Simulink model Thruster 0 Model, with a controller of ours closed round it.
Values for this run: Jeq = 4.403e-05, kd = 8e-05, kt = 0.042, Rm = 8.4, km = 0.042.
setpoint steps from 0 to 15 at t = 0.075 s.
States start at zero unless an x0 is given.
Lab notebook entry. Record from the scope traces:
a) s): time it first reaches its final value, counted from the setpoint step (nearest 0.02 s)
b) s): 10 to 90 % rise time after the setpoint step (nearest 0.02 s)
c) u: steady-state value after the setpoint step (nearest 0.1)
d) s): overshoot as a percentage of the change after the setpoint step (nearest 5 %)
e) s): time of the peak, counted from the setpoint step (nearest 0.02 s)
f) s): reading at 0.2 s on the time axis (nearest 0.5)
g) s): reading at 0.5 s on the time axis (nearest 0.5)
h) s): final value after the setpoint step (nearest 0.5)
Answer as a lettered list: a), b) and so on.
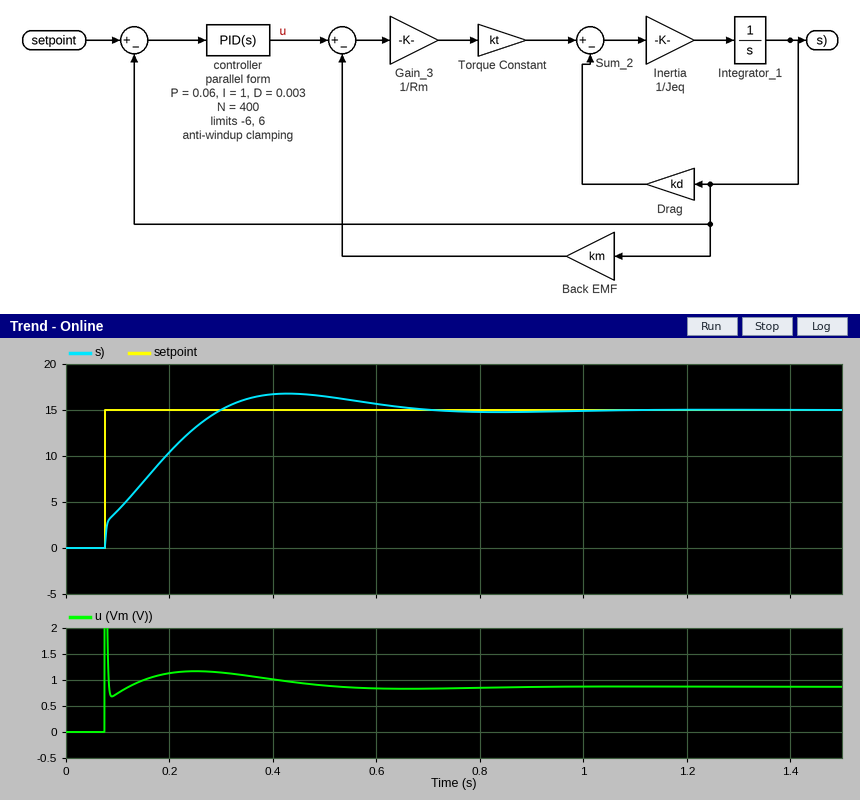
a) 0.22 s
b) 0.18 s
c) 0.9
d) 10 %
e) 0.36 s
f) 10.5
g) 16.5
h) 15.0
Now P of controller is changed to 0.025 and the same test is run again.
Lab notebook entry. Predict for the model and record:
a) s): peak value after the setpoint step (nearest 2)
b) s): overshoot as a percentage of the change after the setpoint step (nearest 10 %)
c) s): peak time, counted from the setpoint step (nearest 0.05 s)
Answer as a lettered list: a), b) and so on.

a) 18
b) 20 %
c) 0.35 s
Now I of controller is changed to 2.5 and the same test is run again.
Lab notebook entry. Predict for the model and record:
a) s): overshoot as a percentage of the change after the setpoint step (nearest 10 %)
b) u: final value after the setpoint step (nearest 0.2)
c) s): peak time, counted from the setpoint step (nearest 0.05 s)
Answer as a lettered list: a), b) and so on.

a) 30 %
b) 0.8
c) 0.20 s
